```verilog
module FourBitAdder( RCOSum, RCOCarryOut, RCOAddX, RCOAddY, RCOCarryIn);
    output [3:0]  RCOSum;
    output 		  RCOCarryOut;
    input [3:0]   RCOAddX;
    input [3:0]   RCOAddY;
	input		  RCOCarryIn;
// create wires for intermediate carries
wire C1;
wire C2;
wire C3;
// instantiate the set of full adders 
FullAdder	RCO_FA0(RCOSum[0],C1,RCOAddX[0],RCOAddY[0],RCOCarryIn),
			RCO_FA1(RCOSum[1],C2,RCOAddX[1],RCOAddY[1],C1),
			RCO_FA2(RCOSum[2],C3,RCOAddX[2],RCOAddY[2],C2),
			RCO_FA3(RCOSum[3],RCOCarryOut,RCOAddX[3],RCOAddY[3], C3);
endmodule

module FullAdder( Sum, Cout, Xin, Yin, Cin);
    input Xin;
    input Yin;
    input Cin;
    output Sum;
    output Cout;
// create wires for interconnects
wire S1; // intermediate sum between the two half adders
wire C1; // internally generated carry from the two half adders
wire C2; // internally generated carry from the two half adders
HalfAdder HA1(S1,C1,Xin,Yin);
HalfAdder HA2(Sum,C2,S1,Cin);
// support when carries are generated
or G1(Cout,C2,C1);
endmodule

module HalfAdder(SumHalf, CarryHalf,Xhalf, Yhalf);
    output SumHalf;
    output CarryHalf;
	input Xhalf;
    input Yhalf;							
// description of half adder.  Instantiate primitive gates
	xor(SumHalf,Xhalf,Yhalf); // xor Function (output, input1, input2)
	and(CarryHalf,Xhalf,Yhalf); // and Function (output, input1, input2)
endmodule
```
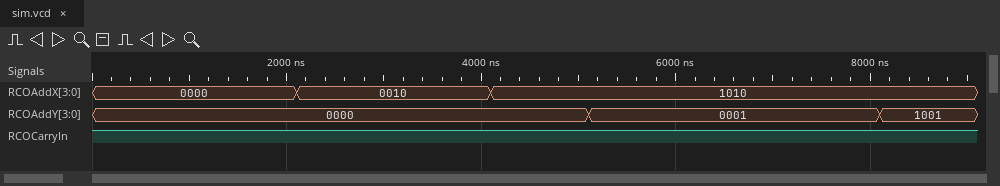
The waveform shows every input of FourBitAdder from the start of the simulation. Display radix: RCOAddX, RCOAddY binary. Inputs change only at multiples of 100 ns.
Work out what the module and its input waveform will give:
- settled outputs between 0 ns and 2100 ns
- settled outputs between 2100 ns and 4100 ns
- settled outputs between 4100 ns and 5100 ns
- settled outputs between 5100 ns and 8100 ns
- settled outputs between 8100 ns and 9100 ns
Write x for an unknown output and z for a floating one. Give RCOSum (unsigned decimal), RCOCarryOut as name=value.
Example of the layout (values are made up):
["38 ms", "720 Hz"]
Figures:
["RCOSum=1, RCOCarryOut=0", "RCOSum=3, RCOCarryOut=0", "RCOSum=11, RCOCarryOut=0", "RCOSum=12, RCOCarryOut=0", "RCOSum=4, RCOCarryOut=1"]
